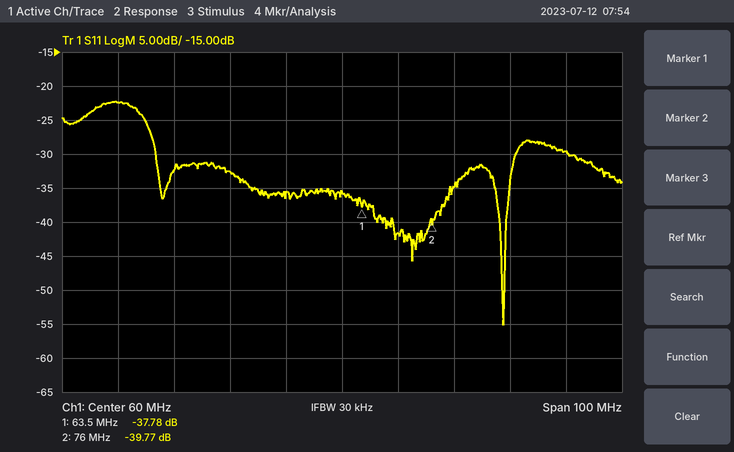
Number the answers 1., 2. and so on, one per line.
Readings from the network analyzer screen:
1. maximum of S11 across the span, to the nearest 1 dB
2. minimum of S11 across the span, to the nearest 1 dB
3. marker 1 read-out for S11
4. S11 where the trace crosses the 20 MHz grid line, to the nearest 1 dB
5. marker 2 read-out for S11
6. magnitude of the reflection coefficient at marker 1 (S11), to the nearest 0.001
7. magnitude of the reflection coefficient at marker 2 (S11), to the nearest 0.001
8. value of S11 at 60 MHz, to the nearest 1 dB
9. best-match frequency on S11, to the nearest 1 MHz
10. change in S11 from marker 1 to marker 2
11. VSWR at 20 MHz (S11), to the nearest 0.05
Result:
1. -22 dB
2. -55 dB
3. -37.78 dB
4. -22 dB
5. -39.77 dB
6. 0.013
7. 0.010
8. -36 dB
9. 89 MHz
10. -1.99 dB
11. 1.15
